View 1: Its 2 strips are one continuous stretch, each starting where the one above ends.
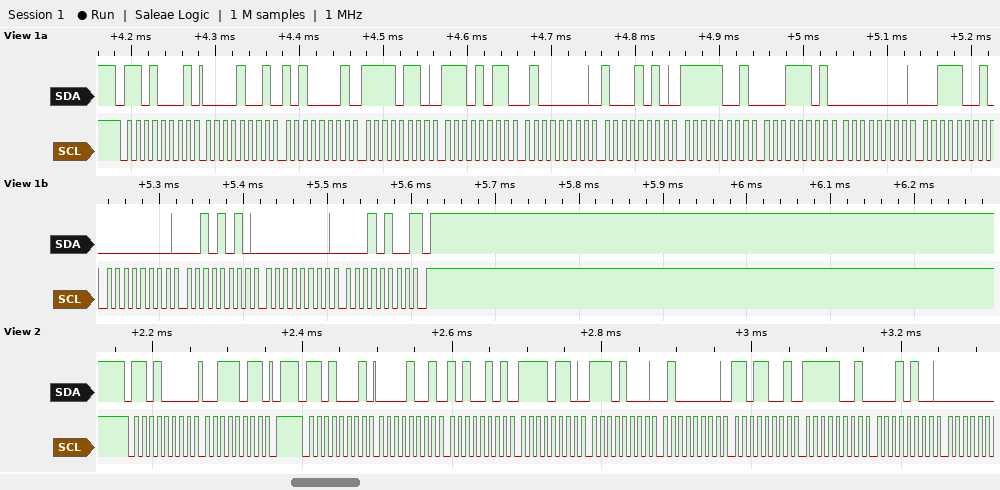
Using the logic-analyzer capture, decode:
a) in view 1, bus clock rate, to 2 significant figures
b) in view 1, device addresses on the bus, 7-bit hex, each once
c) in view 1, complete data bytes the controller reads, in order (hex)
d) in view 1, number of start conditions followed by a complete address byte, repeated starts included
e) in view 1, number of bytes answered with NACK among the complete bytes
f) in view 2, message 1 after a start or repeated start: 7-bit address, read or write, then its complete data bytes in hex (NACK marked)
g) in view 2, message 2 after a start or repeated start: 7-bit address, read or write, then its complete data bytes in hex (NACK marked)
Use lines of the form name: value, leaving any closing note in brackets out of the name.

in view 1, bus clock rate, to 2 significant figures: 100 kHz
in view 1, device addresses on the bus, 7-bit hex, each once: 0x68
in view 1, complete data bytes the controller reads, in order: 09 A1 F6 EB 40 8A F9 1D 00 39 00 2A 00 14
in view 1, number of start conditions followed by a complete address byte, repeated starts included: 1
in view 1, number of bytes answered with NACK among the complete bytes: 1
in view 2, message 1 after a start or repeated start: 7-bit address, read or write, then its complete data bytes in hex: 0x68 write: 3B
in view 2, message 2 after a start or repeated start: 7-bit address, read or write, then its complete data bytes in hex: 0x68 read: 09 A5 F6 E8 40 D9 F9 14
